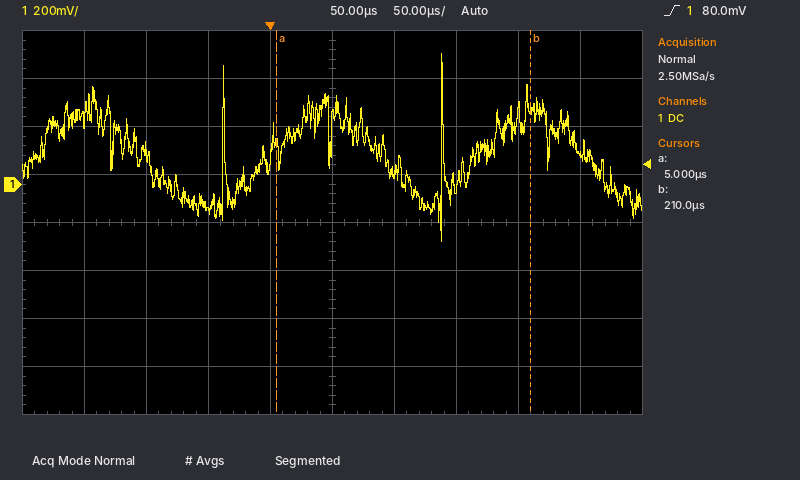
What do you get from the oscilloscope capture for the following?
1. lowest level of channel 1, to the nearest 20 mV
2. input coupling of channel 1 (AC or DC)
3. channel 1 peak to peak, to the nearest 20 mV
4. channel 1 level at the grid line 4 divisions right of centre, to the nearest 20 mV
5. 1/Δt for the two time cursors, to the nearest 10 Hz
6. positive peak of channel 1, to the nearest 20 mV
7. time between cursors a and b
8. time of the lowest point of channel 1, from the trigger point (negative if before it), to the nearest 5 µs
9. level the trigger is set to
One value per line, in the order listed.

-240 mV
DC
780 mV
120 mV
4.88 kHz
540 mV
205 µs
+140 µs
80.0 mV
